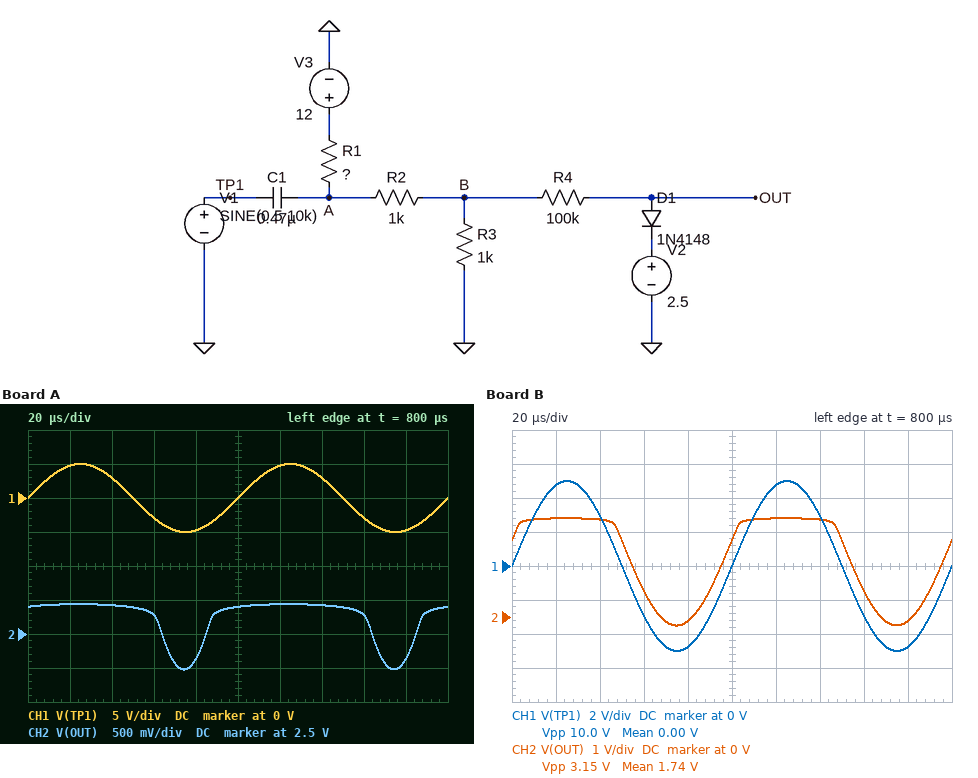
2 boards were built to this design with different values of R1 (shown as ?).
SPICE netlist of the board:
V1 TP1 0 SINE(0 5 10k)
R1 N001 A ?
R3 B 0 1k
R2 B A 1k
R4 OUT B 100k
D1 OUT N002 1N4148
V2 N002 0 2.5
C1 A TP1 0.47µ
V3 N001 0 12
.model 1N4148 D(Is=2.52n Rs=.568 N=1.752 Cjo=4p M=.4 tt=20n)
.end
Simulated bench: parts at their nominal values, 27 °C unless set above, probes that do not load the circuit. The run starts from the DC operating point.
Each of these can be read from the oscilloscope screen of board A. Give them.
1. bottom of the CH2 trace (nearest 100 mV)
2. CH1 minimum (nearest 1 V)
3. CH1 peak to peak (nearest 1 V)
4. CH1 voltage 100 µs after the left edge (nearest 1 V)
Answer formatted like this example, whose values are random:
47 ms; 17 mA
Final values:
2.0 V; -5 V; 10 V; 0 V
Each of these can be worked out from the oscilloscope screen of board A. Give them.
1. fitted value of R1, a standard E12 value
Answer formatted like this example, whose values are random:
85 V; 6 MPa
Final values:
680 Ω
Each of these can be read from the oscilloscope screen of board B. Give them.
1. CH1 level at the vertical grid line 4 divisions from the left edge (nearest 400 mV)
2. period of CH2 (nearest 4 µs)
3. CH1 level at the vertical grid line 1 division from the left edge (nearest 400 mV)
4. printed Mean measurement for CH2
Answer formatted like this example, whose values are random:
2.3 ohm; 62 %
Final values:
-4.8 V; 100 µs; 4.8 V; 1.74 V
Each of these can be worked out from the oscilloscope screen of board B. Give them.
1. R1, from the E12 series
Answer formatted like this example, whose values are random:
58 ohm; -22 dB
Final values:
3.3 kΩ
